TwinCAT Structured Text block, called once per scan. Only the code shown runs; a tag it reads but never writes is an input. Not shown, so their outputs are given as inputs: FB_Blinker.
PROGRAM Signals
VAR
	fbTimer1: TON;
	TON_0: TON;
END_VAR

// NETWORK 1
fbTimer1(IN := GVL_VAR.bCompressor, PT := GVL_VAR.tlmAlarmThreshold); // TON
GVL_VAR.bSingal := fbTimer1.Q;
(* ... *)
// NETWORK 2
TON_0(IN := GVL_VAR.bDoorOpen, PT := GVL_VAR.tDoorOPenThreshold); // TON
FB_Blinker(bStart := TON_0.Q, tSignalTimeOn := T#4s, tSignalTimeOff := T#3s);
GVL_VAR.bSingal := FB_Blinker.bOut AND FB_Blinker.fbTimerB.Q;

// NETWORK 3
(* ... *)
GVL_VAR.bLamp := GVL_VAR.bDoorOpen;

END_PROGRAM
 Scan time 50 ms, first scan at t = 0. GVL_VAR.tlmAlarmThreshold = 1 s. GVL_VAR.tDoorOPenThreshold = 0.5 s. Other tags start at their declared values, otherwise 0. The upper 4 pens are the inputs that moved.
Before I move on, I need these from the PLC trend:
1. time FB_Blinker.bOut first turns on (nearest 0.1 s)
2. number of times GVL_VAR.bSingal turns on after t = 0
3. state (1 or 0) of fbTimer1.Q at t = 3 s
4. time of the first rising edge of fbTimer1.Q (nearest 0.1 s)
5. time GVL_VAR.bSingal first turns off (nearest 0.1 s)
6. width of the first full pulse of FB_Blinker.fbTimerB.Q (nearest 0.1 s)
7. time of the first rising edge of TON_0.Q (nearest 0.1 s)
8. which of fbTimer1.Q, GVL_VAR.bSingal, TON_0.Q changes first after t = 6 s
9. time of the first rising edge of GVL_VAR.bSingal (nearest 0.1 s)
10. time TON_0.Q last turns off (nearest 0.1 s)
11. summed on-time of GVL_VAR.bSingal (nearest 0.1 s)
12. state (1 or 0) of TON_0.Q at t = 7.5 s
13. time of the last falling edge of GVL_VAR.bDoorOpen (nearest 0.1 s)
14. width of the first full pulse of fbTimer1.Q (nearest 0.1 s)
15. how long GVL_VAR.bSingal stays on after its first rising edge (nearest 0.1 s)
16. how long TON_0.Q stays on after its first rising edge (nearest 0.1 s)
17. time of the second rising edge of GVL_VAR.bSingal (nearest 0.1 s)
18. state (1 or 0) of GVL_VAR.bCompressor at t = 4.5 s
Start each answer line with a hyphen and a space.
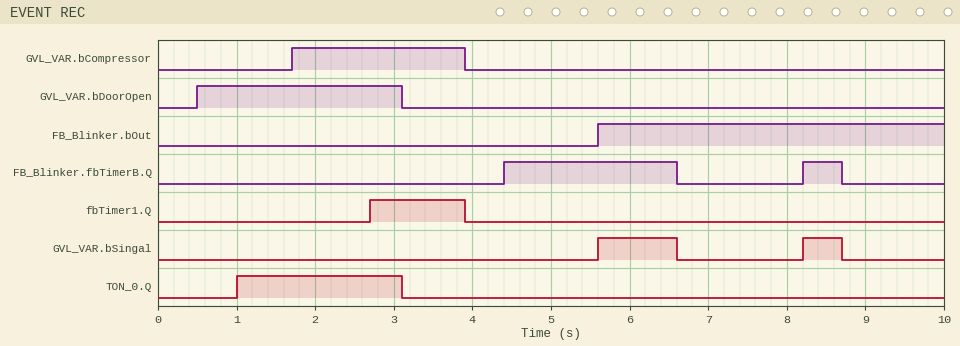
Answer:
- 5.6 s
- 2
- 1
- 2.7 s
- 6.6 s
- 2.2 s
- 1.0 s
- GVL_VAR.bSingal
- 5.6 s
- 3.1 s
- 1.5 s
- 0
- 3.1 s
- 1.2 s
- 1.0 s
- 2.1 s
- 8.2 s
- 0
